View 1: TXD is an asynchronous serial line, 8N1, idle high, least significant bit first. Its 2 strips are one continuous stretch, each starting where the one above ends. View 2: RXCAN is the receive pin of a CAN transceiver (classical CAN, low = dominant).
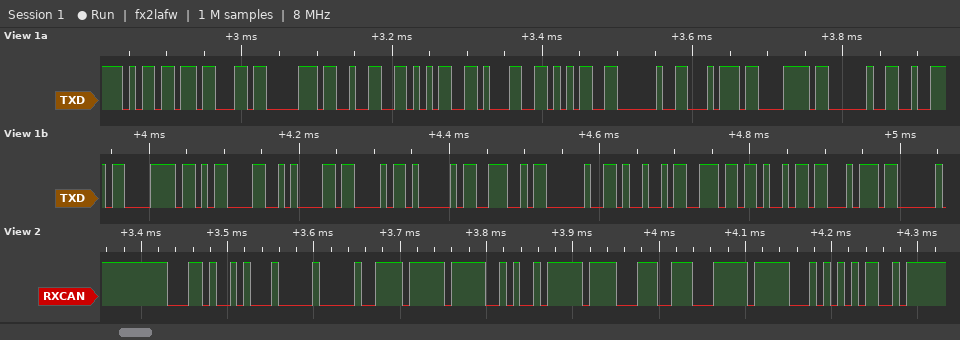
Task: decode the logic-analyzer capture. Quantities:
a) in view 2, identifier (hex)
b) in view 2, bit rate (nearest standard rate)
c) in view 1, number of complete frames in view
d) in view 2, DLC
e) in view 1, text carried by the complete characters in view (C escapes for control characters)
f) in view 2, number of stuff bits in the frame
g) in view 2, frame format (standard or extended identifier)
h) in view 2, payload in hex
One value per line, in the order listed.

0x1A5
125 kbit/s
23
8
"mcp2515 tx rx\r\nCAN Init"
7
standard
00 7B FF 52 FF 8E 71 FF
